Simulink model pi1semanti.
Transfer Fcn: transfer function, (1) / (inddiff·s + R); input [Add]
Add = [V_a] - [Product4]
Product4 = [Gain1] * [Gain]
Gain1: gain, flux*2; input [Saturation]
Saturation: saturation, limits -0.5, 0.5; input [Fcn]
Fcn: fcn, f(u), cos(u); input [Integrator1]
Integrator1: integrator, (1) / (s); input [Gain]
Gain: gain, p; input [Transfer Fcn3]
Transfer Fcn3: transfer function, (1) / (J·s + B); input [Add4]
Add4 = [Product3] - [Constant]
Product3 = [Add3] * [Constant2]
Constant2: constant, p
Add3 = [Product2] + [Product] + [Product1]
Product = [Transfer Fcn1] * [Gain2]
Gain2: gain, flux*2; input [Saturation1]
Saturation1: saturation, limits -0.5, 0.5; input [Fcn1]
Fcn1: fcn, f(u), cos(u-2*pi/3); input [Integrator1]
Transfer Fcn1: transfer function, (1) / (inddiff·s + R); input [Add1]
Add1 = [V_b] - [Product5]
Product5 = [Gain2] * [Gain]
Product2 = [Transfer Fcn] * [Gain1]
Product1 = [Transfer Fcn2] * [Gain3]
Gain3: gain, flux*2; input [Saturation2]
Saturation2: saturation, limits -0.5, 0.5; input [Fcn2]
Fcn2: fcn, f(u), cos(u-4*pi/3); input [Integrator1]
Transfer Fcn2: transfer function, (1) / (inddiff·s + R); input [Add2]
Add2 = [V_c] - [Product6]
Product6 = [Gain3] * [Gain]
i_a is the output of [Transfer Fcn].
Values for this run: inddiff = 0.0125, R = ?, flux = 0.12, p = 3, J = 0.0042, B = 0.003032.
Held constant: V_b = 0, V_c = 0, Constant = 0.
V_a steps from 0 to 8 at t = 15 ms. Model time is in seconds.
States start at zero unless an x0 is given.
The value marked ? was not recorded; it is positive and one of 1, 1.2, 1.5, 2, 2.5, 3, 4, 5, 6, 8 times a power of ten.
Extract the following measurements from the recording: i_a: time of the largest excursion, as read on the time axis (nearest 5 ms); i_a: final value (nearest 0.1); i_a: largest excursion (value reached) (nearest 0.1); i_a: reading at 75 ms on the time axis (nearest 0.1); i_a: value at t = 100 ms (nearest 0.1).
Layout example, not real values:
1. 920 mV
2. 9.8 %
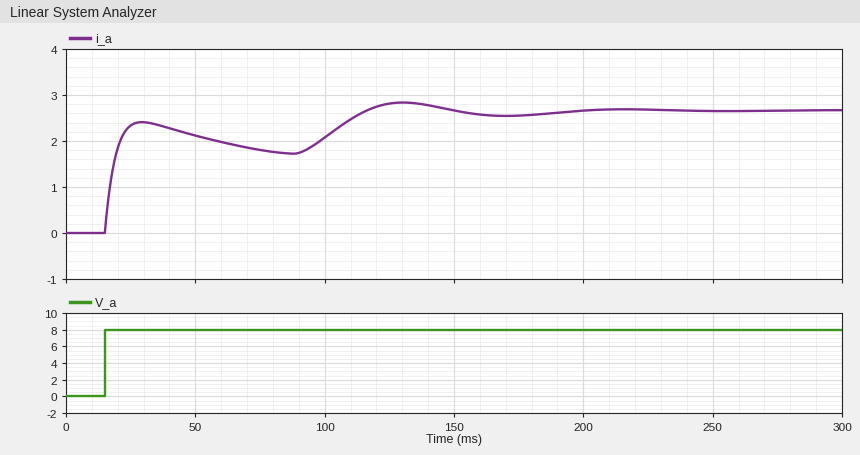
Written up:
1. 130 ms
2. 2.7
3. 2.8
4. 1.8
5. 2.1
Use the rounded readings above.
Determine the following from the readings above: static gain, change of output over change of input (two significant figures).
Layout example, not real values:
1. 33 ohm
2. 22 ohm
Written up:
1. 0.34
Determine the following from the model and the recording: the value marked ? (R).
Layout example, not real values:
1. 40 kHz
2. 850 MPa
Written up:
1. 3
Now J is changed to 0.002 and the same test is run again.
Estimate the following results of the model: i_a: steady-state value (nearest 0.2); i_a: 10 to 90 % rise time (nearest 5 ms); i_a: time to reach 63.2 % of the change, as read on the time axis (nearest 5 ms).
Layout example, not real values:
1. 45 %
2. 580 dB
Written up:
1. 2.6
2. 75 ms
3. 20 ms
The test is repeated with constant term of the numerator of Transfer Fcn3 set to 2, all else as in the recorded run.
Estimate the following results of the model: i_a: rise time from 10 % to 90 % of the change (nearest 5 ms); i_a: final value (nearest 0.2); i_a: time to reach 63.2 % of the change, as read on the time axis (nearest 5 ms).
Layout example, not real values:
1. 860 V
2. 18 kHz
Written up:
1. 75 ms
2. 2.6
3. 20 ms
